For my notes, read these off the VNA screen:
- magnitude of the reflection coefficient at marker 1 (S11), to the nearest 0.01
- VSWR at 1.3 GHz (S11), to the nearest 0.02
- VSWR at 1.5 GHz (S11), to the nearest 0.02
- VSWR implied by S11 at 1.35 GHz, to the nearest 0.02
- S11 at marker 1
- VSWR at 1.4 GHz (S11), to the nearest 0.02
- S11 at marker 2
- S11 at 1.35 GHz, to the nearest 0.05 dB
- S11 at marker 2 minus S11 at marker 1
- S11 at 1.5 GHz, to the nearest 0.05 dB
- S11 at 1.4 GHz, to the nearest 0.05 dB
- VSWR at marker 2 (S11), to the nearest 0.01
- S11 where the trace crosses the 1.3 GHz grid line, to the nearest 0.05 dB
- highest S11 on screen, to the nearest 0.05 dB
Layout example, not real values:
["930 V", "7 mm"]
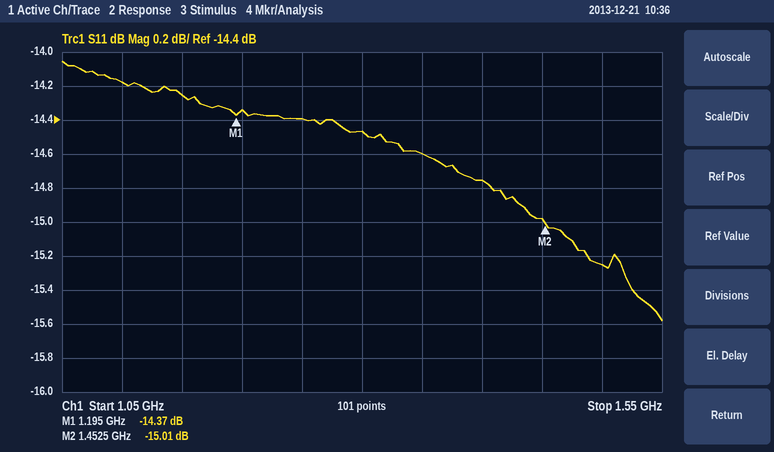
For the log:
["0.19", "1.46", "1.42", "1.46", "-14.37 dB", "1.44", "-15.01 dB", "-14.60 dB", "-0.64 dB", "-15.25 dB", "-14.75 dB", "1.43", "-14.45 dB", "-14.05 dB"]
